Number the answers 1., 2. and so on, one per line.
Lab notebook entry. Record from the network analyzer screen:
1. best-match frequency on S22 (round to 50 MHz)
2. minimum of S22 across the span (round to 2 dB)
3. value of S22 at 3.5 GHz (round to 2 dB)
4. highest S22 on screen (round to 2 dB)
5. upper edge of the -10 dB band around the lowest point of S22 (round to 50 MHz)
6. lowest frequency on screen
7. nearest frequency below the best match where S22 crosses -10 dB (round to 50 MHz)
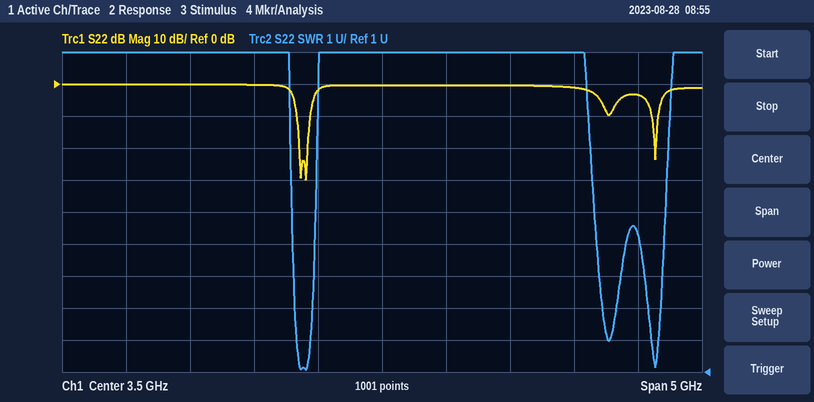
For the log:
1. 2.90 GHz
2. -30 dB
3. 0 dB
4. 0 dB
5. 2.95 GHz
6. 1 GHz
7. 2.85 GHz
